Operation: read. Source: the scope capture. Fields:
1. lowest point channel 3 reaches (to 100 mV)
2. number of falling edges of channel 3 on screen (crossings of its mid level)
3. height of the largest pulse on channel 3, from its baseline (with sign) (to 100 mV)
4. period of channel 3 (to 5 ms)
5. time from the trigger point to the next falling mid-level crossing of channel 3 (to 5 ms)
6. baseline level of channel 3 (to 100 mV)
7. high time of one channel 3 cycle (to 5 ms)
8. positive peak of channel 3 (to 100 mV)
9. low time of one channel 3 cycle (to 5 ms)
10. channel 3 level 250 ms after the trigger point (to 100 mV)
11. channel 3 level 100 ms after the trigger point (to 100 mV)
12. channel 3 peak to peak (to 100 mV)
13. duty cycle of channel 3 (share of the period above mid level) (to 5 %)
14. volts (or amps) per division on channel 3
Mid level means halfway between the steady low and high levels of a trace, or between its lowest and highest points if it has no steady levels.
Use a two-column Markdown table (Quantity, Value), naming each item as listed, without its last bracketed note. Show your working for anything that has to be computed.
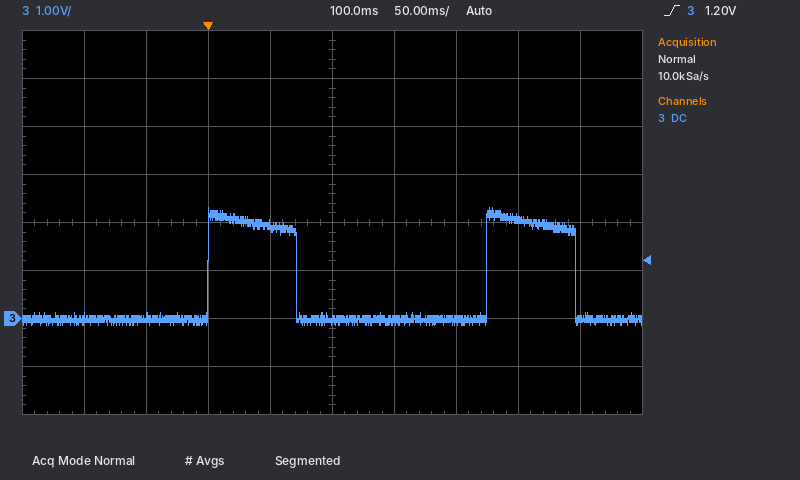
| Quantity | Value |
|---|---|
| lowest point channel 3 reaches | -100 mV |
| number of falling edges of channel 3 on screen | 2 |
| height of the largest pulse on channel 3, from its baseline (with sign) | 2.3 V − (0.0 V) = +2.3 V |
| period of channel 3 | 225 ms |
| time from the trigger point to the next falling mid-level crossing of channel 3 | 70 ms |
| baseline level of channel 3 | 0.0 V |
| high time of one channel 3 cycle | 70 ms |
| positive peak of channel 3 | 2.3 V |
| low time of one channel 3 cycle | 155 ms |
| channel 3 level 250 ms after the trigger point | 2.1 V |
| channel 3 level 100 ms after the trigger point | 0.0 V |
| channel 3 peak to peak | 2.3 V − (-100 mV) = 2.4 V |
| duty cycle of channel 3 (share of the period above mid level) | 70 ms / 225 ms ≈ 31.1 %, so 30 % to the nearest 5 % |
| volts (or amps) per division on channel 3 | 1 V |
